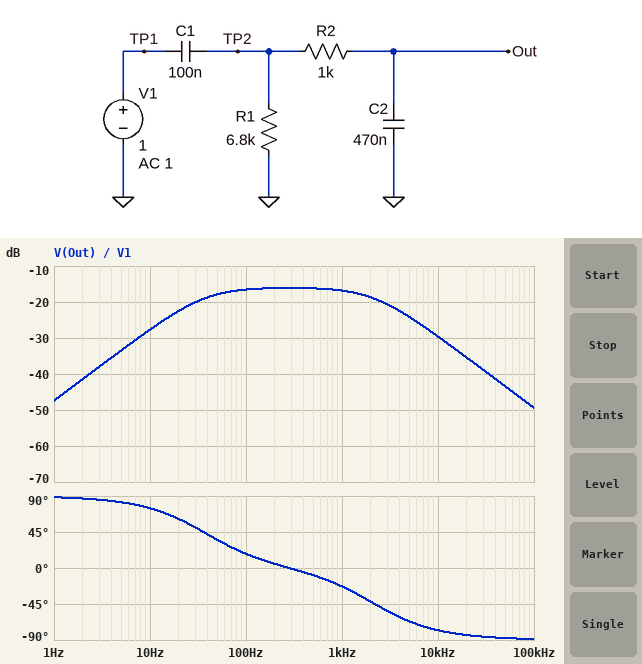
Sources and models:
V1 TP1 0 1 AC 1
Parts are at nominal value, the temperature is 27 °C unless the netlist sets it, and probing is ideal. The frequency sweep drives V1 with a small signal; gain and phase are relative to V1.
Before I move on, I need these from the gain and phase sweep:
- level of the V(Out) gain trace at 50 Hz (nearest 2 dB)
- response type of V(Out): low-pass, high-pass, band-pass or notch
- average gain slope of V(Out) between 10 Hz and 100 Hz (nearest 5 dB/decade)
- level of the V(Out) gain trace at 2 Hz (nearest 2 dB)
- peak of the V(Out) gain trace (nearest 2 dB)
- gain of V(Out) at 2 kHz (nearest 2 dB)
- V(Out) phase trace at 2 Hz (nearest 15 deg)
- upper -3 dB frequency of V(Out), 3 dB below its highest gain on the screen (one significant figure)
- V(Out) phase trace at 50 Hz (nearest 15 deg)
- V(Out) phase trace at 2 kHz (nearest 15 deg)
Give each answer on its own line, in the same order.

-18 dB
band-pass
10 dB/decade
-42 dB
-16 dB
-18 dB
90 deg
2 kHz
30 deg
-45 deg
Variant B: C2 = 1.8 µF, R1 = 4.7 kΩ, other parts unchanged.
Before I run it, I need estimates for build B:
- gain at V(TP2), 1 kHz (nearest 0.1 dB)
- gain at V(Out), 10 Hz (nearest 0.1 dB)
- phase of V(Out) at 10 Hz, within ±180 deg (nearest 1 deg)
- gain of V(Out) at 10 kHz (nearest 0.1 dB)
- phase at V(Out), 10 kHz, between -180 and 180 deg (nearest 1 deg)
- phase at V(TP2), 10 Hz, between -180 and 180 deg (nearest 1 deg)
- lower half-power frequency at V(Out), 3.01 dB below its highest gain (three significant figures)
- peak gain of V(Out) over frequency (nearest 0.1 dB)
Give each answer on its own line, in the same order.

-7.0 dB
-32.2 dB
56 deg
-41.2 dB
-79 deg
62 deg
14.7 Hz
-27.2 dB
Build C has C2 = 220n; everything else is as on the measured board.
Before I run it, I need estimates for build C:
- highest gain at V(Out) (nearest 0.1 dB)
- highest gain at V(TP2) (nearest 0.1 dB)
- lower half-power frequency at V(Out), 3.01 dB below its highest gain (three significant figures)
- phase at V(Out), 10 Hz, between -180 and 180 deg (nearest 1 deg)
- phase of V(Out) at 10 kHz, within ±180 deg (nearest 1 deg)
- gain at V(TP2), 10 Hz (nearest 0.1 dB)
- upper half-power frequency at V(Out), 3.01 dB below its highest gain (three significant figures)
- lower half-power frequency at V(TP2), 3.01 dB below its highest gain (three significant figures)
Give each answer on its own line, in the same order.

-10.9 dB
0 dB
64.8 Hz
81 deg
-76 deg
-27.5 dB
2.61 kHz
2.26 kHz
